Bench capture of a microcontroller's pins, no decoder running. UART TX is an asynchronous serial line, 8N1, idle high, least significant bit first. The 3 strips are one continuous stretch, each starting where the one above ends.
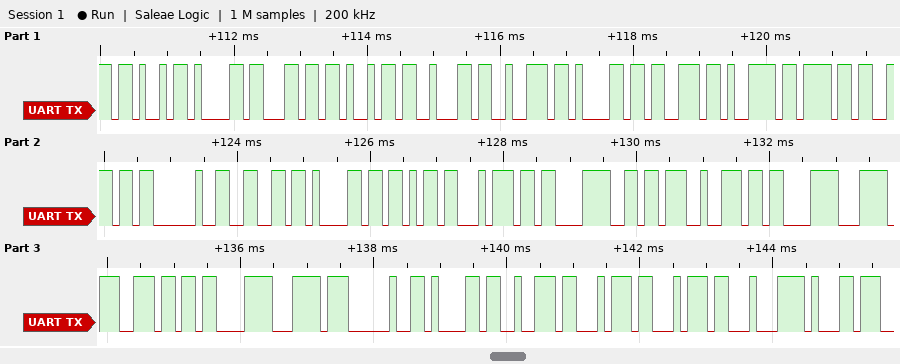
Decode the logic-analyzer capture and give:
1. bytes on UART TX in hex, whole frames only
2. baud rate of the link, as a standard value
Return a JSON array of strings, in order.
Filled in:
["4B 61 6C 69 62 72 61 73 79 6F 6E 20 66 61 6B 74 C3 B6 72 C3 BC 6E C3 BC 20 61 72 74 74 C4 B1", "9600 baud"]
